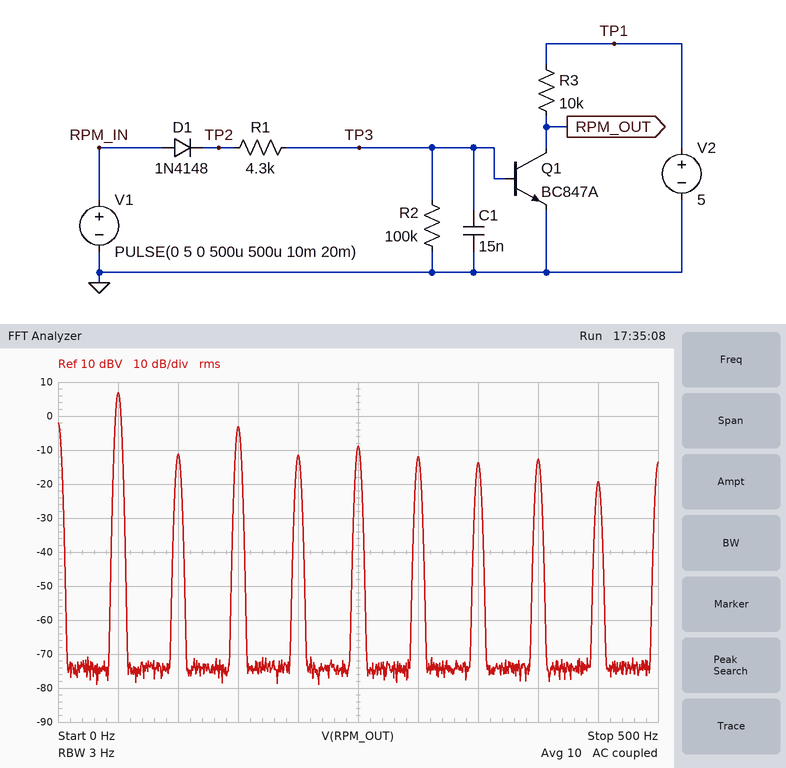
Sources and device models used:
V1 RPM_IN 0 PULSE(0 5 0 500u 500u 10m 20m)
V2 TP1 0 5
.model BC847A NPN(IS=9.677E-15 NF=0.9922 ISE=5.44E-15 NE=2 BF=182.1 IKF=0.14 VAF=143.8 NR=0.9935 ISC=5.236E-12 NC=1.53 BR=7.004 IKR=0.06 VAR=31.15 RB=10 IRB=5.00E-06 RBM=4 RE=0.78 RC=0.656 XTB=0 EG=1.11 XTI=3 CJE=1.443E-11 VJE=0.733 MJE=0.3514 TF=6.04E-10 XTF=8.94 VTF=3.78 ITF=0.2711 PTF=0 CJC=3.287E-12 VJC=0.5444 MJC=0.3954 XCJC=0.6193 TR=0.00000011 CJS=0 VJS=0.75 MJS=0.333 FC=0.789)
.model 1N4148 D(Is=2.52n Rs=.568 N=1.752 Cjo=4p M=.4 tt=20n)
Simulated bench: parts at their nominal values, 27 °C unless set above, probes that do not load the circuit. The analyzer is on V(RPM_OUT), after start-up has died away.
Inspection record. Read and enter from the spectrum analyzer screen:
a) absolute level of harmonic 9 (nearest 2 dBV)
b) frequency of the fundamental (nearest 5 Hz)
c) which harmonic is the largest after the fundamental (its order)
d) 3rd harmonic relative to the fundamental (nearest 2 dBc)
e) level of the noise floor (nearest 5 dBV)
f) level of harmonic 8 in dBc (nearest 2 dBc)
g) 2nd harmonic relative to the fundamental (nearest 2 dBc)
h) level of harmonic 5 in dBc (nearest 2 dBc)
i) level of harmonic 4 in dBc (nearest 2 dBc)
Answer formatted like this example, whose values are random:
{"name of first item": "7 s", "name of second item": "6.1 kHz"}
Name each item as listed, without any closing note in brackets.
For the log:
{"absolute level of harmonic 9": "-20 dBV", "frequency of the fundamental": "50 Hz", "which harmonic is the largest after the fundamental": "3", "3rd harmonic relative to the fundamental": "-10 dBc", "level of the noise floor": "-75 dBV", "level of harmonic 8 in dBc": "-20 dBc", "2nd harmonic relative to the fundamental": "-18 dBc", "level of harmonic 5 in dBc": "-16 dBc", "level of harmonic 4 in dBc": "-18 dBc"}
